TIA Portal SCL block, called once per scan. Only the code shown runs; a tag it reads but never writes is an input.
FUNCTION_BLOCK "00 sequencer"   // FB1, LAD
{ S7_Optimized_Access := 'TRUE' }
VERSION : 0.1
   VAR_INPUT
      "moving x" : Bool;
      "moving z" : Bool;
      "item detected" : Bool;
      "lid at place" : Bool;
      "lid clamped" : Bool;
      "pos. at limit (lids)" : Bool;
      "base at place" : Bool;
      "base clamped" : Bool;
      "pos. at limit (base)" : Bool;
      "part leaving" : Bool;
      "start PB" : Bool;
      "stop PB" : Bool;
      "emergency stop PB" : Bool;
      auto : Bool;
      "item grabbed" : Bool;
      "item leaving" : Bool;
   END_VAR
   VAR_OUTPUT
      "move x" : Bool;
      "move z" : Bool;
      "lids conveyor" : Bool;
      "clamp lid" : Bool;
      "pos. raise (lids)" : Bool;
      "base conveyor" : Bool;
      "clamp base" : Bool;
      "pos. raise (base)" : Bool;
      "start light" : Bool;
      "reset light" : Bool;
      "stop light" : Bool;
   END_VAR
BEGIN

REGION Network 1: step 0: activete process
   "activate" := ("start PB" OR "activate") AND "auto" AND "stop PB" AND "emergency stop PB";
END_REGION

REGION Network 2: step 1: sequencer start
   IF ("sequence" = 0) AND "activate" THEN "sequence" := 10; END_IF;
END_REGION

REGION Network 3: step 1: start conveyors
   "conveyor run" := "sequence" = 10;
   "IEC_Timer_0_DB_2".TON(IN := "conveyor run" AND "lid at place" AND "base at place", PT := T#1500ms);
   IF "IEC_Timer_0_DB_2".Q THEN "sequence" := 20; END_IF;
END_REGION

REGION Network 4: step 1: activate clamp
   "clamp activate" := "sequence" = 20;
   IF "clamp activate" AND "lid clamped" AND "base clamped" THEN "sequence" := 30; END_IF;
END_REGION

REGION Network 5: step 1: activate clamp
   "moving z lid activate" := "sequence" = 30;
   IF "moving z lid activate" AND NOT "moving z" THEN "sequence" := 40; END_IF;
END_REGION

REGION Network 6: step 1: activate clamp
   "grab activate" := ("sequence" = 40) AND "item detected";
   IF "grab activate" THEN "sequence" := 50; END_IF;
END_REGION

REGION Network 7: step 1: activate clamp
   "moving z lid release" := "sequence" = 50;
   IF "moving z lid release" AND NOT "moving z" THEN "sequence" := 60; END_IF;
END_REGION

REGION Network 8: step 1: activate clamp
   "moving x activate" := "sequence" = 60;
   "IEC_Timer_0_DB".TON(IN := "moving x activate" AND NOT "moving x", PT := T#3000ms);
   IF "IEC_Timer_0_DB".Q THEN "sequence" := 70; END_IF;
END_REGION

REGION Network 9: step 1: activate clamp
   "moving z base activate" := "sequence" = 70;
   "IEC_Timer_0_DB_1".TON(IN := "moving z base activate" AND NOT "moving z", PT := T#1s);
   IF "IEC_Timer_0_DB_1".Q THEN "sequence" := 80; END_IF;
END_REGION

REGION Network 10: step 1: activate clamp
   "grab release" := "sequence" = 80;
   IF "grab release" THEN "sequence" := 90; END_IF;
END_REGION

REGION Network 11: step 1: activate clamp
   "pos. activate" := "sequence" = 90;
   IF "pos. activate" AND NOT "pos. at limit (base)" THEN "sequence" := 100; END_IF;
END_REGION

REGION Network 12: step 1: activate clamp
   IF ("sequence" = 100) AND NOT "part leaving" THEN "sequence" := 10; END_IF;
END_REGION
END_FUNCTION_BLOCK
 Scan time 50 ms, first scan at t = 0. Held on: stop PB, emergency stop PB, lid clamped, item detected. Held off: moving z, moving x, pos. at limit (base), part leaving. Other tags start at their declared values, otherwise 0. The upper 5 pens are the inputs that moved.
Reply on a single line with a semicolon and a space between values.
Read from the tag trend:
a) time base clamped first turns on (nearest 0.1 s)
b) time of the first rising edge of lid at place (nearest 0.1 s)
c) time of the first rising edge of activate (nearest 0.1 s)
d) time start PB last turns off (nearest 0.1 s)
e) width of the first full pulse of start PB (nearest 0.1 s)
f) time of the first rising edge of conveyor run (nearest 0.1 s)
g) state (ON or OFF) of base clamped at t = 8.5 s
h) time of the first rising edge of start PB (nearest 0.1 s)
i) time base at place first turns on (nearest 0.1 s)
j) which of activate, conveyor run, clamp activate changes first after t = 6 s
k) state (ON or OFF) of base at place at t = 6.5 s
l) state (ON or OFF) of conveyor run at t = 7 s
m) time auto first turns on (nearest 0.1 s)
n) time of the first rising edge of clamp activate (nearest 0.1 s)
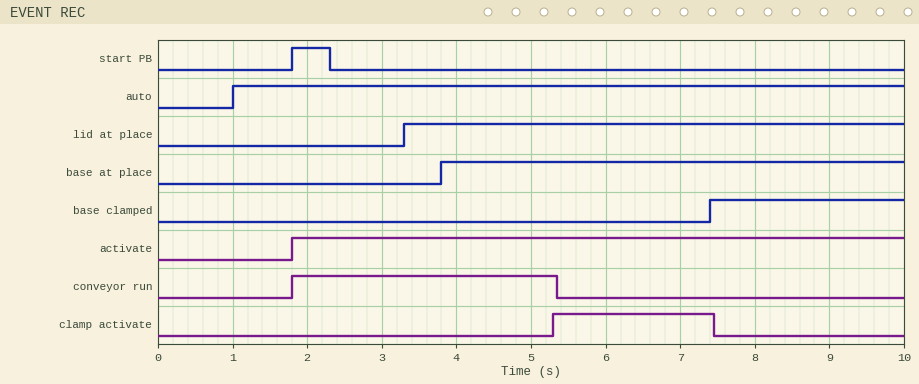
7.4 s; 3.3 s; 1.8 s; 2.3 s; 0.5 s; 1.8 s; ON; 1.8 s; 3.8 s; clamp activate; ON; OFF; 1.0 s; 5.3 s
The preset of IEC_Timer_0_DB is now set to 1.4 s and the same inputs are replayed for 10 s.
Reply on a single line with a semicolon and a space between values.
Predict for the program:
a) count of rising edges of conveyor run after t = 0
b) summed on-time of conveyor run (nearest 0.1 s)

2; 3.7 s
